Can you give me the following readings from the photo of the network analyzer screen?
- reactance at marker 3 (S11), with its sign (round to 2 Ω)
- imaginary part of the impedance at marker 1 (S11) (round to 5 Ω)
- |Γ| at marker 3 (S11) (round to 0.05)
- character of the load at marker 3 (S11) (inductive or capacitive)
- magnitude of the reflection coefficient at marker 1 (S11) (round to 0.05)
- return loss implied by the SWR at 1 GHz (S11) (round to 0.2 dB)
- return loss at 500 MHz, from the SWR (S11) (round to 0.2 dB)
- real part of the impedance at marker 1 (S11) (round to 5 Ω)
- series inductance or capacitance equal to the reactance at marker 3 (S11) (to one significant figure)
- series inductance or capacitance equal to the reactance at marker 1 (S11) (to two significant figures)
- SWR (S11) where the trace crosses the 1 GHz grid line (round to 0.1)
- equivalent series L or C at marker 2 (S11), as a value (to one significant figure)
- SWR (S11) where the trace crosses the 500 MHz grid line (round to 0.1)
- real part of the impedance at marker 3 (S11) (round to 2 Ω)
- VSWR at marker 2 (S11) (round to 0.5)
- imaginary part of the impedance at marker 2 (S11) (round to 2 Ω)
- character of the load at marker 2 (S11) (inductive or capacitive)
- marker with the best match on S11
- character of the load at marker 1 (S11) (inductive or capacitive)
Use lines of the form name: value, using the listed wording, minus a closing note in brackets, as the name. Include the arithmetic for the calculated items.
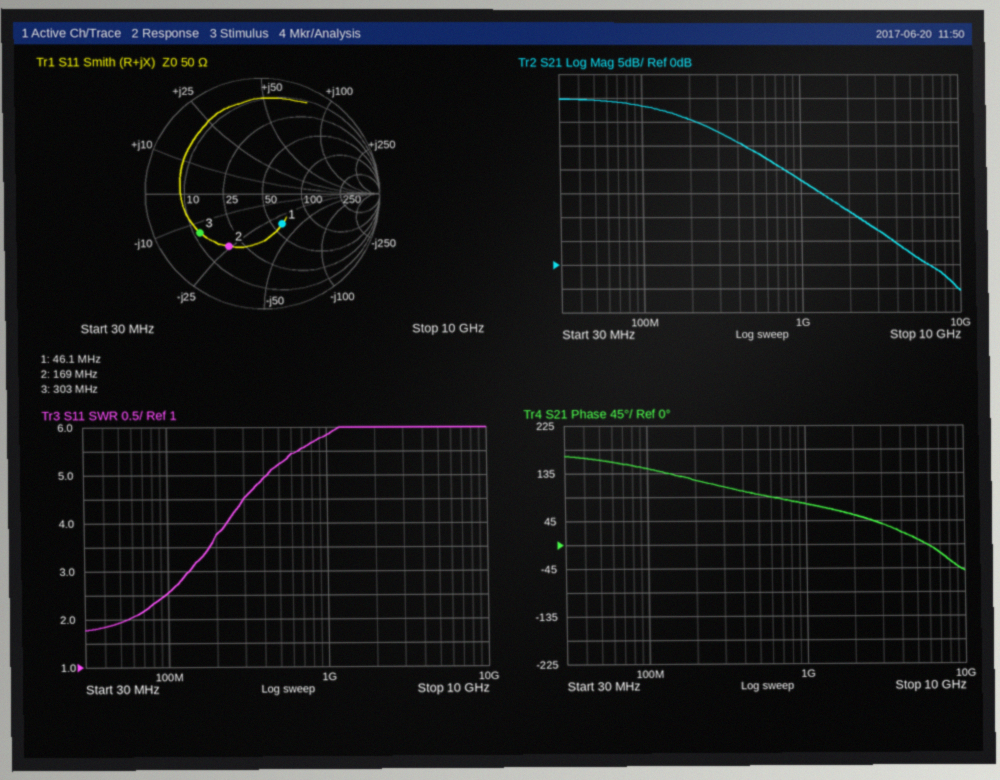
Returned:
reactance at marker 3 (S11), with its sign: -14 Ω
imaginary part of the impedance at marker 1 (S11): -35 Ω
|Γ| at marker 3 (S11): 0.65
character of the load at marker 3 (S11): capacitive
magnitude of the reflection coefficient at marker 1 (S11): 0.30
return loss implied by the SWR at 1 GHz (S11): −20 log10((5.8 − 1)/(5.8 + 1)) ≈ 3.0 dB
return loss at 500 MHz, from the SWR (S11): −20 log10((5.2 − 1)/(5.2 + 1)) ≈ 3.4 dB
real part of the impedance at marker 1 (S11): 60 Ω
series inductance or capacitance equal to the reactance at marker 3 (S11): C = 1/(2π × 303 MHz × 14 Ω) ≈ 37.5 pF, so 40 pF to one significant figure
series inductance or capacitance equal to the reactance at marker 1 (S11): C = 1/(2π × 46.1 MHz × 35 Ω) ≈ 98.6 pF, so 100 pF to two significant figures
SWR (S11) where the trace crosses the 1 GHz grid line: 5.8
equivalent series L or C at marker 2 (S11), as a value: C = 1/(2π × 169 MHz × 24 Ω) ≈ 39.2 pF, so 40 pF to one significant figure
SWR (S11) where the trace crosses the 500 MHz grid line: 5.2
real part of the impedance at marker 3 (S11): 12 Ω
VSWR at marker 2 (S11): 3.5
imaginary part of the impedance at marker 2 (S11): -24 Ω
character of the load at marker 2 (S11): capacitive
marker with the best match on S11: marker 1
character of the load at marker 1 (S11): capacitive
